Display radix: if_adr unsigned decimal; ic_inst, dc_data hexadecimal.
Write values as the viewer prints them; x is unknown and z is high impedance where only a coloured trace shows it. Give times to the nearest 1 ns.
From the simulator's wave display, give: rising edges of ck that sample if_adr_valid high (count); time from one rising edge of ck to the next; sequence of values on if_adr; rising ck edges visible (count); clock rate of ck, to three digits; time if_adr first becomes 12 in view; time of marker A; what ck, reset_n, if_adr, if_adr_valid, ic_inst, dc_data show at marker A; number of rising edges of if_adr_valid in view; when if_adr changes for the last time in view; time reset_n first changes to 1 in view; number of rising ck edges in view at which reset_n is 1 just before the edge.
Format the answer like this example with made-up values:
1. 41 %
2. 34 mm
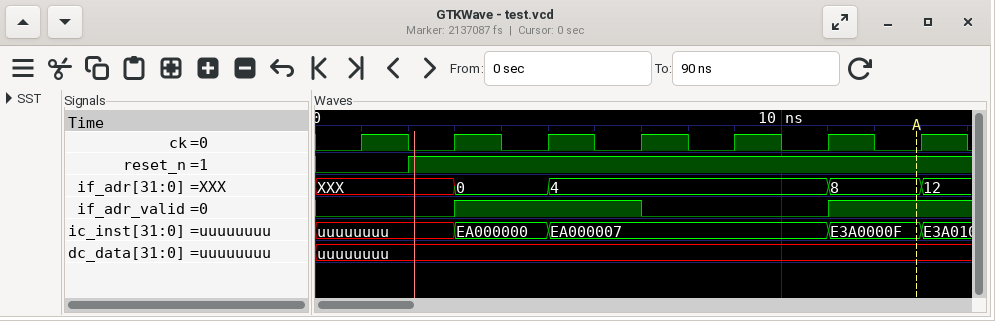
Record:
1. 3
2. 2 ns
3. XXX, 0, 4, 8, 12
4. 7
5. 500 MHz
6. 13 ns
7. 13 ns
8. ck=0, reset_n=1, if_adr=8, if_adr_valid=1, ic_inst=E3A0000F, dc_data=uuuuuuuu
9. 2
10. 13 ns
11. 2 ns
12. 6
